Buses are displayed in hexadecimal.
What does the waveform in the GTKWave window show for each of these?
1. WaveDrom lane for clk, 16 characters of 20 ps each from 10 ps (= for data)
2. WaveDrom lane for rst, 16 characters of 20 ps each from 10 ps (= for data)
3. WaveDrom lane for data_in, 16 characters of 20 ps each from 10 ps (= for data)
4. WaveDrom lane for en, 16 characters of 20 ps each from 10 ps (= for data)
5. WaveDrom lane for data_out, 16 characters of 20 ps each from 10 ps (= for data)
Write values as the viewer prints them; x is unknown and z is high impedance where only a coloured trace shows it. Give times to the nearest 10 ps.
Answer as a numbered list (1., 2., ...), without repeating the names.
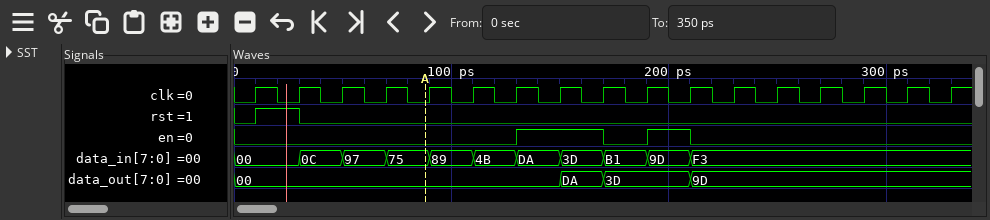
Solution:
1. {name: 'clk', wave: 'p...............'}
2. {name: 'rst', wave: '10..............'}
3. {name: 'data_in', wave: '===========.....', data: '00 0C 97 75 89 4B DA 3D B1 9D F3'}
4. {name: 'en', wave: '0.....1.010.....'}
5. {name: 'data_out', wave: '=......==.=.....', data: '00 DA 3D 9D'}
